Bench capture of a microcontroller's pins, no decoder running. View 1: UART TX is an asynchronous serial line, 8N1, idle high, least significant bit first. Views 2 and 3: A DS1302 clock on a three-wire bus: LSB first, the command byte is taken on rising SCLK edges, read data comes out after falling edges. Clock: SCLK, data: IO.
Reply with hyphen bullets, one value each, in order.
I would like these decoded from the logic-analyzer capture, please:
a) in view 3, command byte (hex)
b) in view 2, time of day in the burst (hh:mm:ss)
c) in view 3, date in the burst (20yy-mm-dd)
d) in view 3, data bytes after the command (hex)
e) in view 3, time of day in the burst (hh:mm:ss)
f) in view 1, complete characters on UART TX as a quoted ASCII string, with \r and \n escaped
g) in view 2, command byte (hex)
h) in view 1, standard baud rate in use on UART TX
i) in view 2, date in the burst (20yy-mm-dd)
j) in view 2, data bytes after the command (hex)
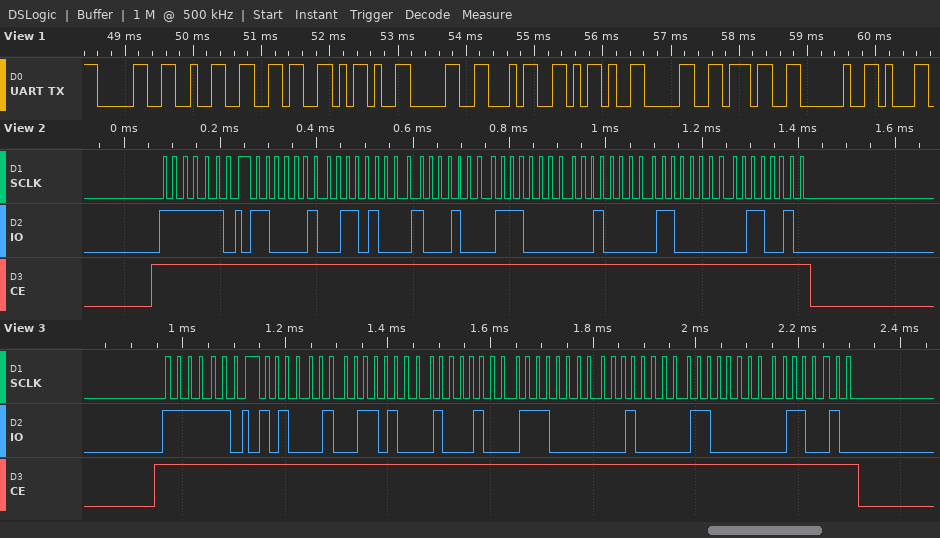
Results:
- 0xBF
- 11:16:43
- 2026-04-07
- 45 16 11 07 04 03 26
- 11:16:45
- "026-04-07 "
- 0xBF
- 9600 baud
- 2026-04-07
- 43 16 11 07 04 03 26
